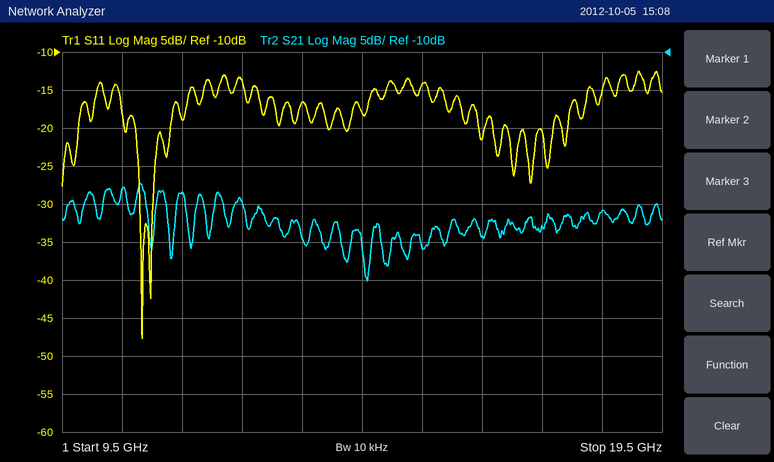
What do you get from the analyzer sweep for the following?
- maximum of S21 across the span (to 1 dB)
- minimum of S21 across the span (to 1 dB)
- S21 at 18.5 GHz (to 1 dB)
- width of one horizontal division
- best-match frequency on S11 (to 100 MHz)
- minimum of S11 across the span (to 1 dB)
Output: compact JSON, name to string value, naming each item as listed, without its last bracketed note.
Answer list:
{"maximum of S21 across the span": "-27 dB", "minimum of S21 across the span": "-40 dB", "S21 at 18.5 GHz": "-31 dB", "width of one horizontal division": "1 GHz", "best-match frequency on S11": "10.8 GHz", "minimum of S11 across the span": "-48 dB"}
